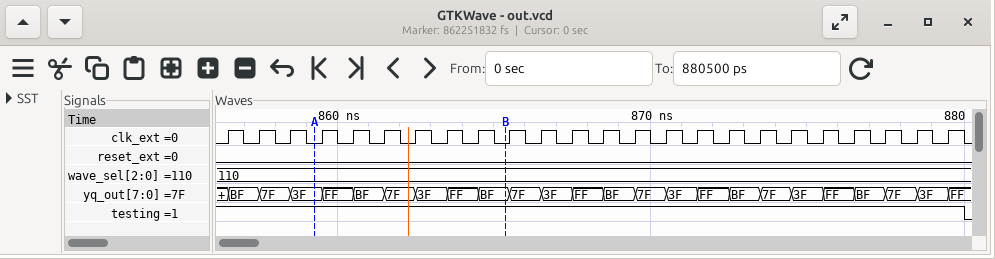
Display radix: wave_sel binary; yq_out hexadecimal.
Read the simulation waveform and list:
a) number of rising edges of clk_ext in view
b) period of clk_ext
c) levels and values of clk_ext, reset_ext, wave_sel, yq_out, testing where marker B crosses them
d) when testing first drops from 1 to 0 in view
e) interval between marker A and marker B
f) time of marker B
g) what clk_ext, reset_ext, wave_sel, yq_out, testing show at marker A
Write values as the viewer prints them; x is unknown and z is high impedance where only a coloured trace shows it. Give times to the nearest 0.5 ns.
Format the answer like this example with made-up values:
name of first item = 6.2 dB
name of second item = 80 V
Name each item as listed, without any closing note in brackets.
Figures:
number of rising edges of clk_ext in view = 24
period of clk_ext = 1 ns
levels and values of clk_ext, reset_ext, wave_sel, yq_out, testing where marker B crosses them = clk_ext=0, reset_ext=0, wave_sel=110, yq_out=BF, testing=1
when testing first drops from 1 to 0 in view = 880 ns
interval between marker A and marker B = 6 ns
time of marker B = 865.5 ns
what clk_ext, reset_ext, wave_sel, yq_out, testing show at marker A = clk_ext=0, reset_ext=0, wave_sel=110, yq_out=3F, testing=1
